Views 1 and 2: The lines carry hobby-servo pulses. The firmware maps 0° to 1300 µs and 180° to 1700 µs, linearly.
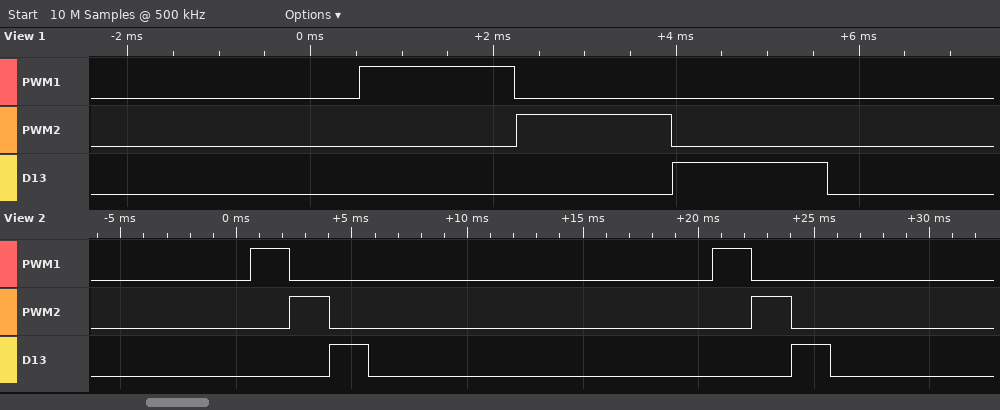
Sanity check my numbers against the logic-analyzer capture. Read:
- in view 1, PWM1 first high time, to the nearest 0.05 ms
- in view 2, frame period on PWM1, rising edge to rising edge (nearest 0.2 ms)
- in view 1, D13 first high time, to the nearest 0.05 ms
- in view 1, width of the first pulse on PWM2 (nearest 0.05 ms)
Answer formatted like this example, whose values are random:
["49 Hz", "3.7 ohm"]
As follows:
["1.70 ms", "20.0 ms", "1.70 ms", "1.70 ms"]
